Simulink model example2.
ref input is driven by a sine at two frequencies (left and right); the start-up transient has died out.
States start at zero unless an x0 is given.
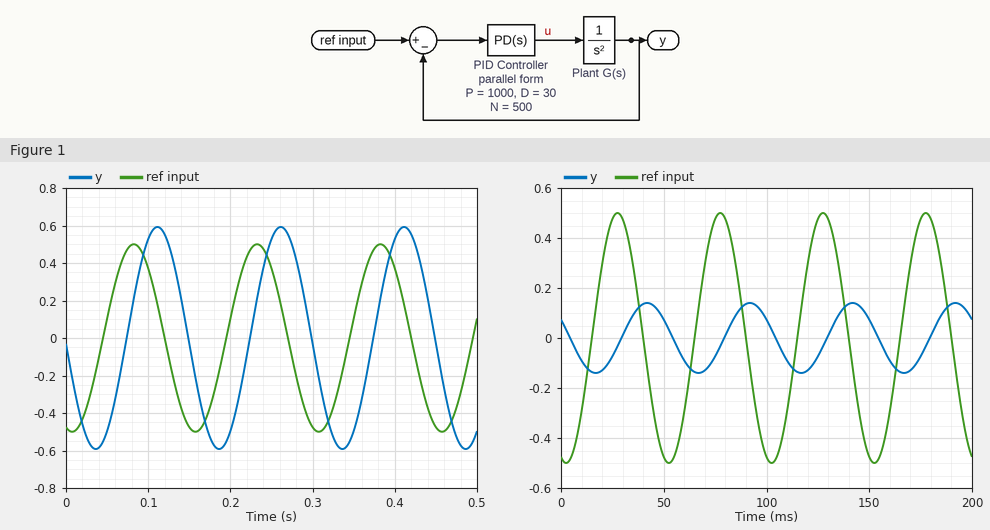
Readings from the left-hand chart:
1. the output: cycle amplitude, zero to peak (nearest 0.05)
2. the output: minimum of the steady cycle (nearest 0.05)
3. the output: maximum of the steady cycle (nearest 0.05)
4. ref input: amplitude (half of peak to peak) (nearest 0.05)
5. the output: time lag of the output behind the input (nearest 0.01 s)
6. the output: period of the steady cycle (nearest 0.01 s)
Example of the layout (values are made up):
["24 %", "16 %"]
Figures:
["0.60", "-0.60", "0.60", "0.50", "0.03 s", "0.15 s"]
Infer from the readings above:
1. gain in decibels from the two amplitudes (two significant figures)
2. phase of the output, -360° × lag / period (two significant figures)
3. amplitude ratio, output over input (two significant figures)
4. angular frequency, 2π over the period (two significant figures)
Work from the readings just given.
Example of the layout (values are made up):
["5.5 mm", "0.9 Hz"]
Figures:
["1.6 dB", "-72°", "1.2", "42 rad/s"]
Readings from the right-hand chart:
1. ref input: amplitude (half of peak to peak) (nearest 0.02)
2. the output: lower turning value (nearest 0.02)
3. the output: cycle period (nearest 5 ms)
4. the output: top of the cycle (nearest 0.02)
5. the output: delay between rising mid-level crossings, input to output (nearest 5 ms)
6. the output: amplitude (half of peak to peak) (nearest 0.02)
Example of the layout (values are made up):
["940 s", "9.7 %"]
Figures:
["0.50", "-0.14", "50 ms", "0.14", "15 ms", "0.14"]
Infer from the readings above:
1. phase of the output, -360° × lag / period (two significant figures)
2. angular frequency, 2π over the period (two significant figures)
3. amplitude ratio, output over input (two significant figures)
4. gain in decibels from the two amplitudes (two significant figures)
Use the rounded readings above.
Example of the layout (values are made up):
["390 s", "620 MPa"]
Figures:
["-110°", "0.13 rad/ms", "0.28", "-11 dB"]
